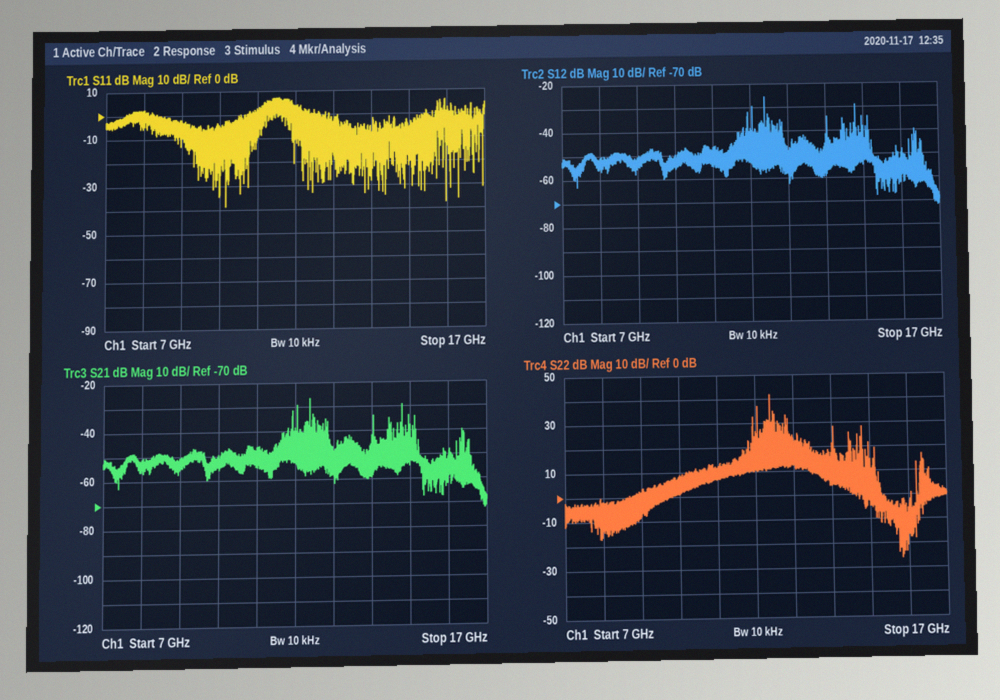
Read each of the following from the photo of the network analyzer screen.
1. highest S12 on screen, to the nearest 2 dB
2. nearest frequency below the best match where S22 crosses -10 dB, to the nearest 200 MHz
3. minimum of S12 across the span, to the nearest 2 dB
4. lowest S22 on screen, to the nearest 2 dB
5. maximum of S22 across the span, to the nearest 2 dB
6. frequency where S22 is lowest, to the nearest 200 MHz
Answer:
-26 dB
15.8 GHz
-72 dB
-26 dB
42 dB
15.8 GHz
